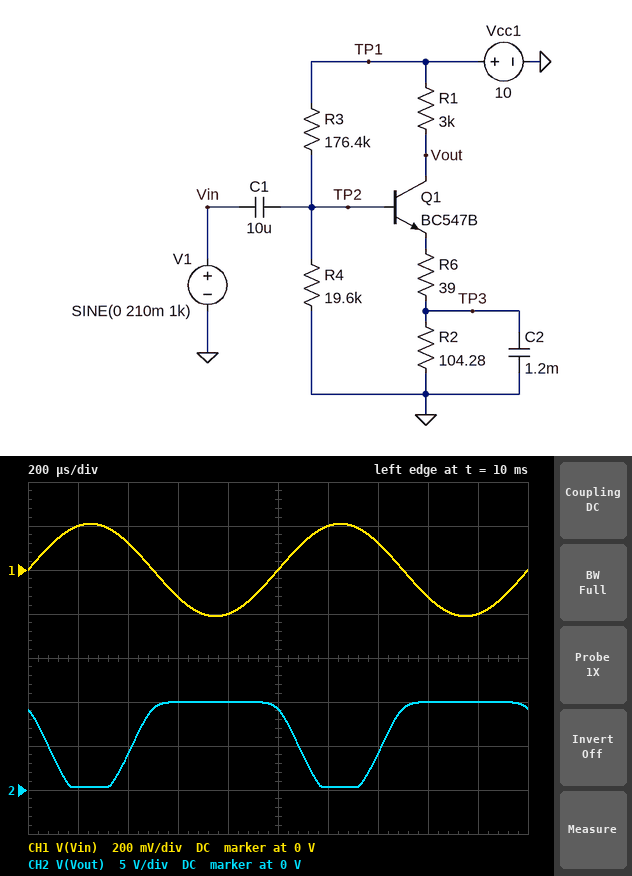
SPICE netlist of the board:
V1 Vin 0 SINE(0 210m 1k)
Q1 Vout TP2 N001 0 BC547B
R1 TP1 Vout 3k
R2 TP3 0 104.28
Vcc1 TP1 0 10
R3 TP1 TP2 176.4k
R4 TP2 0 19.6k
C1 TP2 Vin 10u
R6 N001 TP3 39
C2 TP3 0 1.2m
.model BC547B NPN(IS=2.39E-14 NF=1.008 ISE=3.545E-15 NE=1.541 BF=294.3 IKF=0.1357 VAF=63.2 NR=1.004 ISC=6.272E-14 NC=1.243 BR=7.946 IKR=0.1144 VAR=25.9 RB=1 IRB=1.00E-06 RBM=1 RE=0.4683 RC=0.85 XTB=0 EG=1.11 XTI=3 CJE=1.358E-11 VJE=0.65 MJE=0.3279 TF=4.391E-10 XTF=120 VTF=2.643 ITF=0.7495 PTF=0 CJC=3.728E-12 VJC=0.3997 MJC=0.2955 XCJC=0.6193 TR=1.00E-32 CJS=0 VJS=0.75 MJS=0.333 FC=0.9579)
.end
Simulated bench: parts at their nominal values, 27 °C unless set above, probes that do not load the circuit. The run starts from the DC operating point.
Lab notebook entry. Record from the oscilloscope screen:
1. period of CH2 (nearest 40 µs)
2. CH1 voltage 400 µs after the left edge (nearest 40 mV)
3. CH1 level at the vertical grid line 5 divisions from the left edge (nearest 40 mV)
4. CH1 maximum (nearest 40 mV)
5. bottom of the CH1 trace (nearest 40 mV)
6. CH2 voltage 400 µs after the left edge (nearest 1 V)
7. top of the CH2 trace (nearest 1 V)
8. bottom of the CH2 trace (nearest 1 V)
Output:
1.00 ms
120 mV
0 V
200 mV
-200 mV
4 V
10 V
0 V
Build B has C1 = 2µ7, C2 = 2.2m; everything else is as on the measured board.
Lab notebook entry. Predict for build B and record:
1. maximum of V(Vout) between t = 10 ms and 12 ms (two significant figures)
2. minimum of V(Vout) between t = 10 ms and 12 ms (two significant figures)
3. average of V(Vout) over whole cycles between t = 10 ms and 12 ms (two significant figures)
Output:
10 V
360 mV
6.9 V
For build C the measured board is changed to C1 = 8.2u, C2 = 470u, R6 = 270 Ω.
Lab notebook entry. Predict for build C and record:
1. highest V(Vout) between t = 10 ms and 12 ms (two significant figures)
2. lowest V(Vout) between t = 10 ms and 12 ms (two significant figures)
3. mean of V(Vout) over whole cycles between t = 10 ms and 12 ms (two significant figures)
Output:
9.4 V
5.3 V
7.4 V
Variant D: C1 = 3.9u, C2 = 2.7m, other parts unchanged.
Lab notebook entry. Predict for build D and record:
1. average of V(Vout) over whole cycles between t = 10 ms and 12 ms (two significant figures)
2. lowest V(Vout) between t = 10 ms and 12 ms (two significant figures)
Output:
6.9 V
360 mV
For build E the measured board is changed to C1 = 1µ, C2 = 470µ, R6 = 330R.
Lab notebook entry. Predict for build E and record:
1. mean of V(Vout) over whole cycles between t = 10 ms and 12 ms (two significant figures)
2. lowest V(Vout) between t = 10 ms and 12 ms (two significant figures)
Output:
7.7 V
6.0 V
